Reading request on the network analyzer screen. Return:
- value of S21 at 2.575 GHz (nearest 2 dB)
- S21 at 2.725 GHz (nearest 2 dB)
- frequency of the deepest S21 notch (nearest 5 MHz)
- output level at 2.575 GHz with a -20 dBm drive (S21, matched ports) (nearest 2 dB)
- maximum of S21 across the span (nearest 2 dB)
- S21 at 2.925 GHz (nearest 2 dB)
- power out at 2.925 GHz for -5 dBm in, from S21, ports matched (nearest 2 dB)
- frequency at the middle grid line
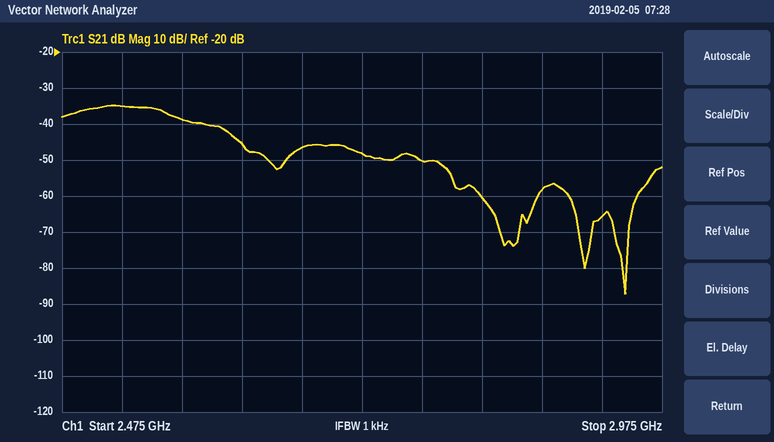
-38 dB
-48 dB
2.945 GHz
-58 dBm
-34 dB
-66 dB
-70 dBm
2.725 GHz
